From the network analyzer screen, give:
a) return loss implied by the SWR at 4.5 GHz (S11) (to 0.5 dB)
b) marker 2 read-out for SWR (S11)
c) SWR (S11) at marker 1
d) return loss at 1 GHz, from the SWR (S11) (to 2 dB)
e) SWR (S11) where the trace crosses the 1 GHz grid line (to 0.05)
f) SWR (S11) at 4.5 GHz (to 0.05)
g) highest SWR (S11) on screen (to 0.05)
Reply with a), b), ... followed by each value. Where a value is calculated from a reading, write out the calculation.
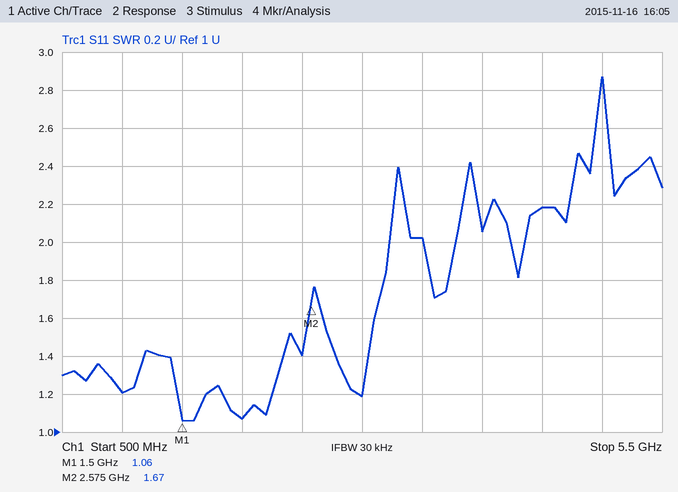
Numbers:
a) −20 log10((2.2 − 1)/(2.2 + 1)) ≈ 8.5 dB
b) 1.67
c) 1.06
d) −20 log10((1.2 − 1)/(1.2 + 1)) ≈ 20.8 dB, so 20 dB to the nearest 2 dB
e) 1.20
f) 2.20
g) 2.85
